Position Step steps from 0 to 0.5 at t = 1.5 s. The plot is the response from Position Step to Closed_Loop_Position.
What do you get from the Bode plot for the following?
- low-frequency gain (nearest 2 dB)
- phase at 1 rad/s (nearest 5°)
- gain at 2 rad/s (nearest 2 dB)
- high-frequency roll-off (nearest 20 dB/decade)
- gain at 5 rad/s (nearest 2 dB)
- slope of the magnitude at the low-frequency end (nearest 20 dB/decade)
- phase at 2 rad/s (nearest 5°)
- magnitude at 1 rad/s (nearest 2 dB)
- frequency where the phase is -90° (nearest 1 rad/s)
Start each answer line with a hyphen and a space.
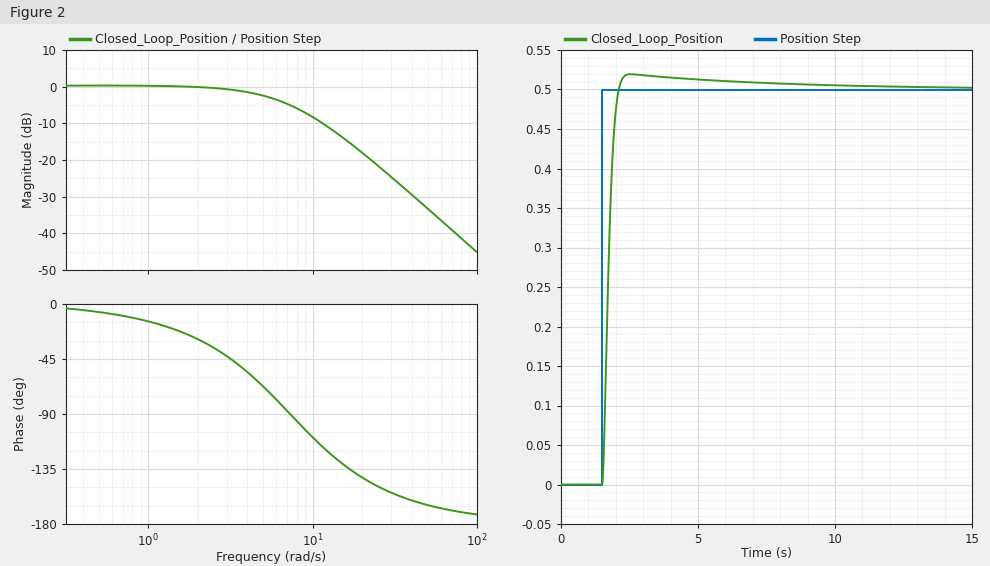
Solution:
- 0 dB
- -15°
- 0 dB
- -40 dB/decade
- -2 dB
- 0 dB/decade
- -30°
- 0 dB
- 7 rad/s
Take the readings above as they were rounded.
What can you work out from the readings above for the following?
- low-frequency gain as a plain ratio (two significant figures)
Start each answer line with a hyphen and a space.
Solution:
- 1.0
